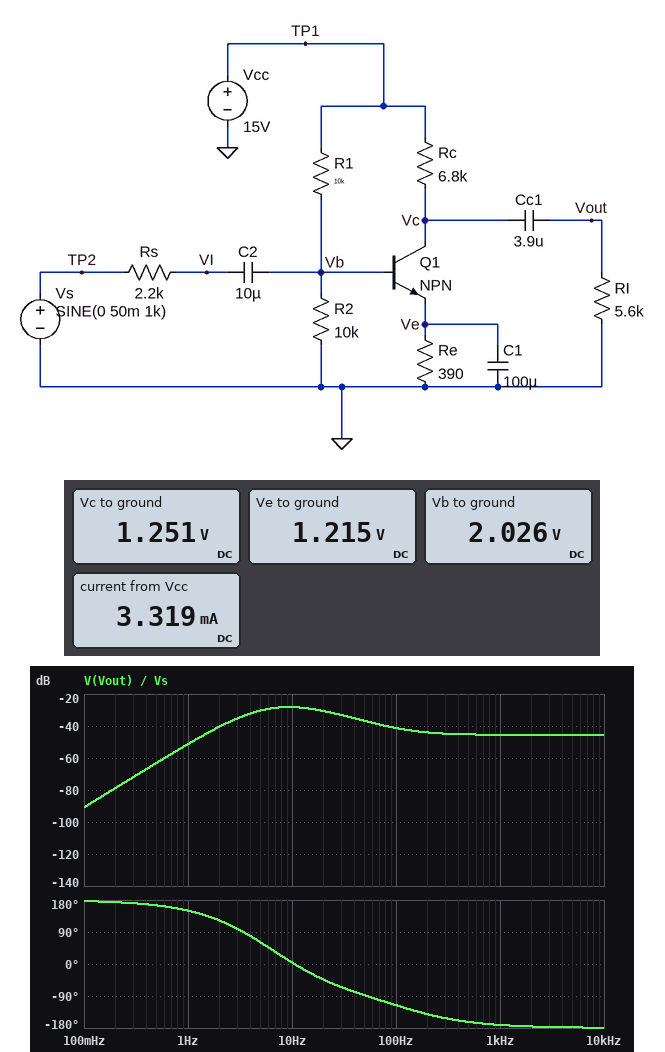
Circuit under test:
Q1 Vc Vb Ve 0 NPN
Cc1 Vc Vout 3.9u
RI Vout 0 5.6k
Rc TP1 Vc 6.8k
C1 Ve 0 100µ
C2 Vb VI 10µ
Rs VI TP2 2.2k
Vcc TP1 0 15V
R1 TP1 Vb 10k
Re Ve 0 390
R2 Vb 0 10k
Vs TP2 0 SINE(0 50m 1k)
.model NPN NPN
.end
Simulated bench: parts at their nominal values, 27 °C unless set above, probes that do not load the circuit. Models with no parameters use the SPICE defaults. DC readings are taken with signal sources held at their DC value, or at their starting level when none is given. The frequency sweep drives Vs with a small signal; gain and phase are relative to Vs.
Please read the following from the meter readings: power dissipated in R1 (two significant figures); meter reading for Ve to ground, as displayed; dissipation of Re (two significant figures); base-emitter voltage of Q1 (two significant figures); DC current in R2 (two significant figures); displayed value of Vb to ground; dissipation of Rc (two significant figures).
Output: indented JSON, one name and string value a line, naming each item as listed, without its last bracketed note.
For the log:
{
  "power dissipated in R1": "17 mW",
  "meter reading for Ve to ground, as displayed": "1.215 V",
  "dissipation of Re": "3.8 mW",
  "base-emitter voltage of Q1": "810 mV",
  "DC current in R2": "200 µA",
  "displayed value of Vb to ground": "2.026 V",
  "dissipation of Rc": "28 mW"
}
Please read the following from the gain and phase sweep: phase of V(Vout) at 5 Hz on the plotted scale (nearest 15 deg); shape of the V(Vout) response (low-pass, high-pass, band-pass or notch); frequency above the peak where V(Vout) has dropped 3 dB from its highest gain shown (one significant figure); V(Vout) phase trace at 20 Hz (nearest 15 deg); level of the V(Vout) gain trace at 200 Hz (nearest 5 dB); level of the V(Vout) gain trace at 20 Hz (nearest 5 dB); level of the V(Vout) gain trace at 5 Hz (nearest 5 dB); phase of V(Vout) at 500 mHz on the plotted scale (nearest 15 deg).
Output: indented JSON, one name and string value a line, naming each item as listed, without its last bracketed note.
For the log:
{
  "phase of V(Vout) at 5 Hz on the plotted scale": "60 deg",
  "shape of the V(Vout) response": "band-pass",
  "frequency above the peak where V(Vout) has dropped 3 dB from its highest gain shown": "20 Hz",
  "V(Vout) phase trace at 20 Hz": "-45 deg",
  "level of the V(Vout) gain trace at 200 Hz": "-45 dB",
  "level of the V(Vout) gain trace at 20 Hz": "-30 dB",
  "level of the V(Vout) gain trace at 5 Hz": "-30 dB",
  "phase of V(Vout) at 500 mHz on the plotted scale": "165 deg"
}
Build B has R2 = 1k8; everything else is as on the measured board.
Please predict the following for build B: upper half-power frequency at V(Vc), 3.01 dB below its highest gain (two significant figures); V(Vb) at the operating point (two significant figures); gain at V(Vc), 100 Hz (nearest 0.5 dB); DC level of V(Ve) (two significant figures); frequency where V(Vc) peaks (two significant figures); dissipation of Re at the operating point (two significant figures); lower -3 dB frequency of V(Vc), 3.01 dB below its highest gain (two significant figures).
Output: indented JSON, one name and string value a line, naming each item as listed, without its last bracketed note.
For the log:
{
  "upper half-power frequency at V(Vc), 3.01 dB below its highest gain": "25 Hz",
  "V(Vb) at the operating point": "1.7 V",
  "gain at V(Vc), 100 Hz": "-31.5 dB",
  "DC level of V(Ve)": "940 mV",
  "frequency where V(Vc) peaks": "6.8 Hz",
  "dissipation of Re at the operating point": "2.3 mW",
  "lower -3 dB frequency of V(Vc), 3.01 dB below its highest gain": "2.5 Hz"
}
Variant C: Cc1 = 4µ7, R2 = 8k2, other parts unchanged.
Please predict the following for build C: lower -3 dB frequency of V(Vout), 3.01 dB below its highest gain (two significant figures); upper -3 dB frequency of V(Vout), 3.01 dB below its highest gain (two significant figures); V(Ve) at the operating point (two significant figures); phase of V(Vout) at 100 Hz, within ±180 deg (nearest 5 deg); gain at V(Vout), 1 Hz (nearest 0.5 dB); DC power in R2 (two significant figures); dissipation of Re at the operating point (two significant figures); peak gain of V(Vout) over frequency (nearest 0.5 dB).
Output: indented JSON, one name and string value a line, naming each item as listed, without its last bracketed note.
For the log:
{
  "lower -3 dB frequency of V(Vout), 3.01 dB below its highest gain": "4.2 Hz",
  "upper -3 dB frequency of V(Vout), 3.01 dB below its highest gain": "21 Hz",
  "V(Ve) at the operating point": "1.2 V",
  "phase of V(Vout) at 100 Hz, within ±180 deg": "-120 deg",
  "gain at V(Vout), 1 Hz": "-50.0 dB",
  "DC power in R2": "490 µW",
  "dissipation of Re at the operating point": "3.7 mW",
  "peak gain of V(Vout) over frequency": "-27.5 dB"
}
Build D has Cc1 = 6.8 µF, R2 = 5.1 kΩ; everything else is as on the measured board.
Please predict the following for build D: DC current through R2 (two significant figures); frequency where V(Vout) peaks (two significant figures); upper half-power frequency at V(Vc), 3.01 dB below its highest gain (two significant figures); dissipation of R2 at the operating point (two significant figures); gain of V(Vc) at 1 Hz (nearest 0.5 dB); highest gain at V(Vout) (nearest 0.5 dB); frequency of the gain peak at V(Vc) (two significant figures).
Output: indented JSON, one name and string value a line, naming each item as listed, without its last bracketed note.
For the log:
{
  "DC current through R2": "380 µA",
  "frequency where V(Vout) peaks": "7.9 Hz",
  "upper half-power frequency at V(Vc), 3.01 dB below its highest gain": "16 Hz",
  "dissipation of R2 at the operating point": "750 µW",
  "gain of V(Vc) at 1 Hz": "-34.5 dB",
  "highest gain at V(Vout)": "-27.0 dB",
  "frequency of the gain peak at V(Vc)": "6.0 Hz"
}
